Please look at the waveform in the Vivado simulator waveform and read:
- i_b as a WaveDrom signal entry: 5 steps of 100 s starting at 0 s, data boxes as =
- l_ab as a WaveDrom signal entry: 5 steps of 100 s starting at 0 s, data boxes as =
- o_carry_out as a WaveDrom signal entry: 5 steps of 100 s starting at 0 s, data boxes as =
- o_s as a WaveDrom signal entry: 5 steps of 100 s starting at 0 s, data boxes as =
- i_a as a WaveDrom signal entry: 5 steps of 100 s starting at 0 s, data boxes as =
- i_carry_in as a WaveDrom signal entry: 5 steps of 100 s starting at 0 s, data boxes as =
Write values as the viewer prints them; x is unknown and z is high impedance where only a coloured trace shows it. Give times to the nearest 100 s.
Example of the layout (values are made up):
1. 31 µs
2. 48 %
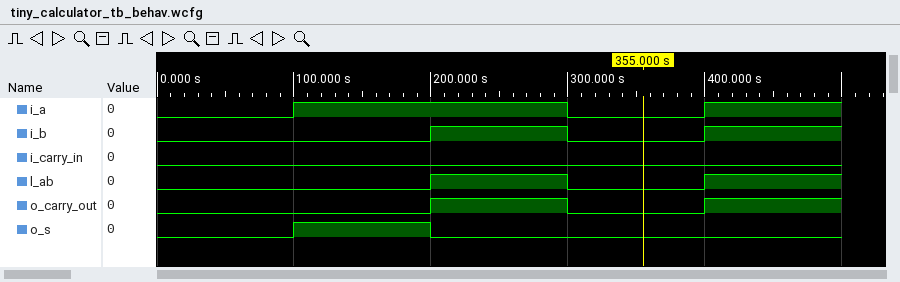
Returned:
1. {name: 'i_b', wave: '0.101'}
2. {name: 'l_ab', wave: '0.101'}
3. {name: 'o_carry_out', wave: '0.101'}
4. {name: 'o_s', wave: '010..'}
5. {name: 'i_a', wave: '01.01'}
6. {name: 'i_carry_in', wave: '0....'}
